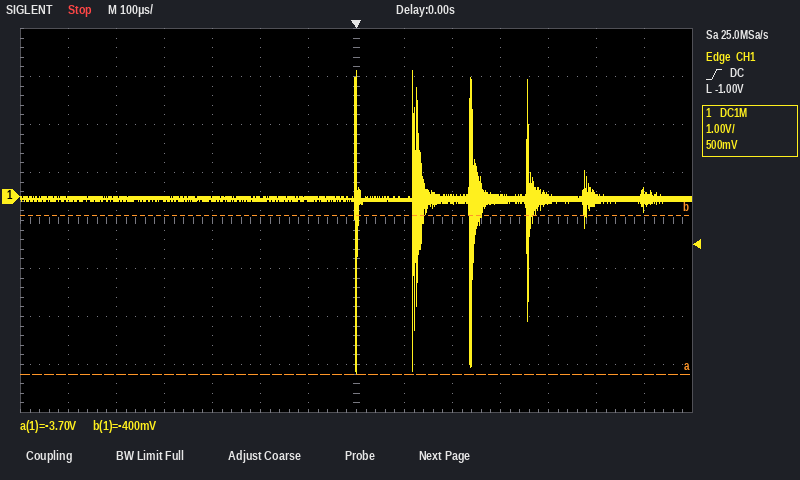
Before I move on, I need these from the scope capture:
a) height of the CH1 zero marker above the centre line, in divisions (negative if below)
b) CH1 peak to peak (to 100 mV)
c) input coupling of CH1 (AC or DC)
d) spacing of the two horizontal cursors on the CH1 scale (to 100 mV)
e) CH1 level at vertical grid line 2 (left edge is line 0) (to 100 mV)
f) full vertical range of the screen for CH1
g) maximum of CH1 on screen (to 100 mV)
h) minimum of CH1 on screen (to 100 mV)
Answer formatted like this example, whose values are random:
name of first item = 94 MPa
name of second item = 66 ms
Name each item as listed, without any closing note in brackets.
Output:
height of the CH1 zero marker above the centre line, in divisions = +0.5 div
CH1 peak to peak = 6.3 V
input coupling of CH1 = DC
spacing of the two horizontal cursors on the CH1 scale = 3.3 V
CH1 level at vertical grid line 2 (left edge is line 0) = 0.0 V
full vertical range of the screen for CH1 = 8 V
maximum of CH1 on screen = 2.6 V
minimum of CH1 on screen = -3.7 V
